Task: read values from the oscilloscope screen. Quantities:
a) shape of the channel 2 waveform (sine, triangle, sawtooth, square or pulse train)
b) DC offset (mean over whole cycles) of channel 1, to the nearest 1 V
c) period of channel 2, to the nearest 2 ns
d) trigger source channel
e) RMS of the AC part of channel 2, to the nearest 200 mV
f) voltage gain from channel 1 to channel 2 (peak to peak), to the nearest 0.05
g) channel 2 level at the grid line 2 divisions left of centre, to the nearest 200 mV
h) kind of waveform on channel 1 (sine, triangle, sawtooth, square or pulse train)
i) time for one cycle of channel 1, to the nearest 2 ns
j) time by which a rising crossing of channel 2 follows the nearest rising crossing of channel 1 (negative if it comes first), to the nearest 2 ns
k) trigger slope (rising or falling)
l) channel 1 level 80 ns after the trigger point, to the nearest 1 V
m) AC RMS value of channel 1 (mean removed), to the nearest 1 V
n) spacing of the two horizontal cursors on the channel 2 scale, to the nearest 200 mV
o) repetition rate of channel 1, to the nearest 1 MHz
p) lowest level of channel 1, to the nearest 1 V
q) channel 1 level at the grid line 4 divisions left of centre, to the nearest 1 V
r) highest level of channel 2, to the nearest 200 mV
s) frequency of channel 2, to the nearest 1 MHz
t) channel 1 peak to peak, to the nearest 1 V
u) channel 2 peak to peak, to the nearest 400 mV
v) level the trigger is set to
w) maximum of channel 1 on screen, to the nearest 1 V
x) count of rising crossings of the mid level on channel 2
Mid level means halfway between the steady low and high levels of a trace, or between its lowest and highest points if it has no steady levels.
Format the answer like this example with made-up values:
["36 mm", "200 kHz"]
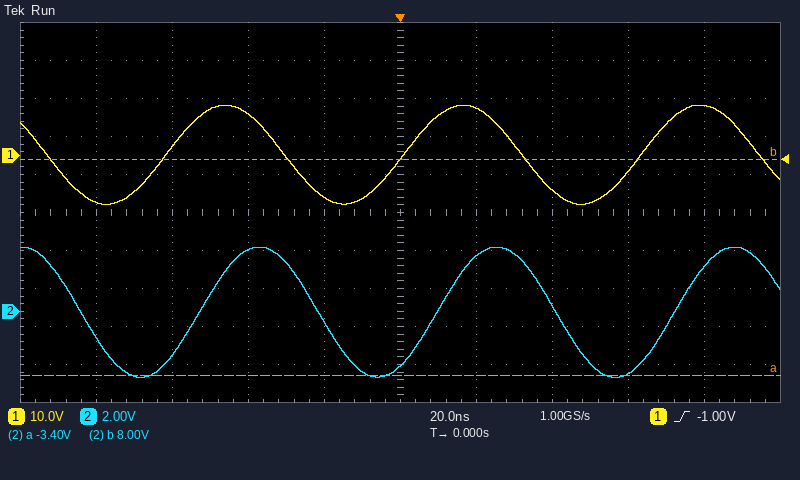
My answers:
["sine", "0 V", "62 ns", "channel 1", "2.4 V", "0.25", "3.2 V", "sine", "62 ns", "+8 ns", "rising", "13 V", "9 V", "11.4 V", "16 MHz", "-13 V", "-12 V", "3.4 V", "16 MHz", "26 V", "6.8 V", "-1.00 V", "13 V", "3"]
